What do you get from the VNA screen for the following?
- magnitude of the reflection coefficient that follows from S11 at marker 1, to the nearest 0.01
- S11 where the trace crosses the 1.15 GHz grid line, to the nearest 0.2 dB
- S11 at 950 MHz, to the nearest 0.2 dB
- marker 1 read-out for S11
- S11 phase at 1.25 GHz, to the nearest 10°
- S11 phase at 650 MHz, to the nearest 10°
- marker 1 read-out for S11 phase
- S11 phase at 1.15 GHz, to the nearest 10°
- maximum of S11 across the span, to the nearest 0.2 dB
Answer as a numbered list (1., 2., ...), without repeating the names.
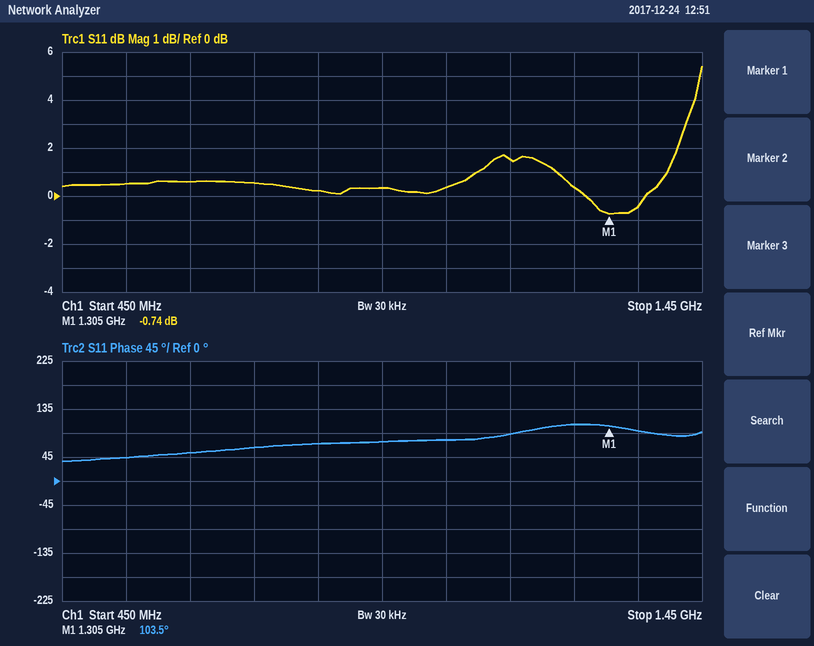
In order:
1. 0.92
2. 1.6 dB
3. 0.4 dB
4. -0.74 dB
5. 110°
6. 50°
7. 103.5°
8. 90°
9. 5.4 dB
